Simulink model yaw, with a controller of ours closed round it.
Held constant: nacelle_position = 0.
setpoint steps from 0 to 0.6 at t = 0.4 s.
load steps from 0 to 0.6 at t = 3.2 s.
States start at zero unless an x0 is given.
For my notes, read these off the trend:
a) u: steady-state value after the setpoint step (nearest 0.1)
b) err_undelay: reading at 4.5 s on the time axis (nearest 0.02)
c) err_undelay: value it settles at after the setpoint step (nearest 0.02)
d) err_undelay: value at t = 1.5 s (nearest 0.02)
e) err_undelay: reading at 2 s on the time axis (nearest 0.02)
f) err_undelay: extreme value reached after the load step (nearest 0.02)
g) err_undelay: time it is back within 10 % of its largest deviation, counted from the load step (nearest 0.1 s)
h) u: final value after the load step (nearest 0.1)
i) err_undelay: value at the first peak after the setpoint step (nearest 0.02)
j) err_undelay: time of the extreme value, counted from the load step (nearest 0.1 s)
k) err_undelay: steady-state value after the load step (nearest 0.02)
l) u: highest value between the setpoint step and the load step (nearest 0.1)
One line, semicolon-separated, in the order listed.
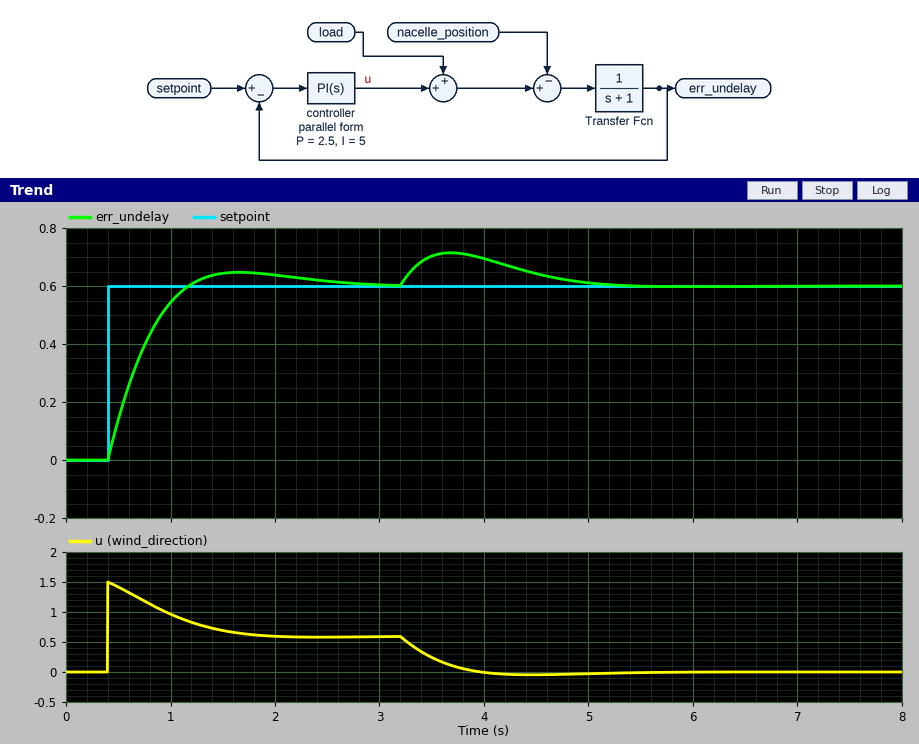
0.6; 0.64; 0.60; 0.64; 0.64; 0.72; 1.8 s; 0.0; 0.64; 0.5 s; 0.60; 1.5
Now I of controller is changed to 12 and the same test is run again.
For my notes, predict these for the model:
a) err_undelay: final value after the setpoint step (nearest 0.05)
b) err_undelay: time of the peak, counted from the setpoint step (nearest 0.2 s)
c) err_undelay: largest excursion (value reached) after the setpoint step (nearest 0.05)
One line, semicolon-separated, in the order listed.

0.60; 0.8 s; 0.75
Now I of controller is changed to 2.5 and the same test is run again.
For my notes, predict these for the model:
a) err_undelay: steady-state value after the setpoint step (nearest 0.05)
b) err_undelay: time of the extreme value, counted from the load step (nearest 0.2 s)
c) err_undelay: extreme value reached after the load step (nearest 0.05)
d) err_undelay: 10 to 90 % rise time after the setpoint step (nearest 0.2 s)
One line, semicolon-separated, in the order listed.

0.60; 0.6 s; 0.75; 0.8 s
